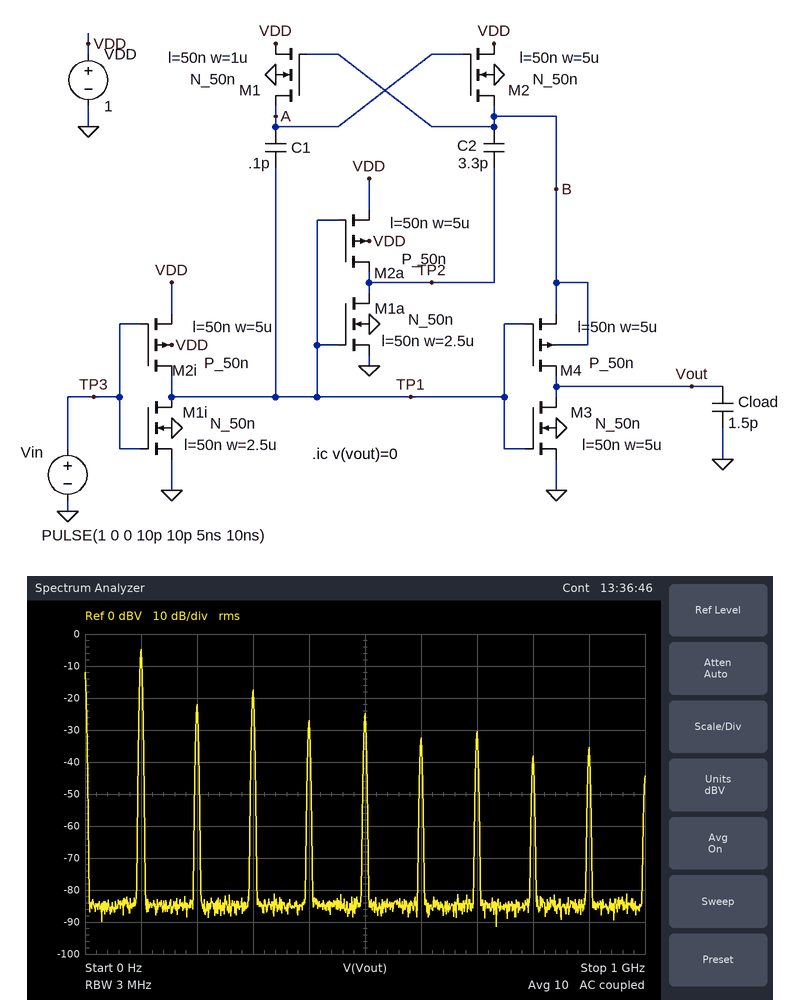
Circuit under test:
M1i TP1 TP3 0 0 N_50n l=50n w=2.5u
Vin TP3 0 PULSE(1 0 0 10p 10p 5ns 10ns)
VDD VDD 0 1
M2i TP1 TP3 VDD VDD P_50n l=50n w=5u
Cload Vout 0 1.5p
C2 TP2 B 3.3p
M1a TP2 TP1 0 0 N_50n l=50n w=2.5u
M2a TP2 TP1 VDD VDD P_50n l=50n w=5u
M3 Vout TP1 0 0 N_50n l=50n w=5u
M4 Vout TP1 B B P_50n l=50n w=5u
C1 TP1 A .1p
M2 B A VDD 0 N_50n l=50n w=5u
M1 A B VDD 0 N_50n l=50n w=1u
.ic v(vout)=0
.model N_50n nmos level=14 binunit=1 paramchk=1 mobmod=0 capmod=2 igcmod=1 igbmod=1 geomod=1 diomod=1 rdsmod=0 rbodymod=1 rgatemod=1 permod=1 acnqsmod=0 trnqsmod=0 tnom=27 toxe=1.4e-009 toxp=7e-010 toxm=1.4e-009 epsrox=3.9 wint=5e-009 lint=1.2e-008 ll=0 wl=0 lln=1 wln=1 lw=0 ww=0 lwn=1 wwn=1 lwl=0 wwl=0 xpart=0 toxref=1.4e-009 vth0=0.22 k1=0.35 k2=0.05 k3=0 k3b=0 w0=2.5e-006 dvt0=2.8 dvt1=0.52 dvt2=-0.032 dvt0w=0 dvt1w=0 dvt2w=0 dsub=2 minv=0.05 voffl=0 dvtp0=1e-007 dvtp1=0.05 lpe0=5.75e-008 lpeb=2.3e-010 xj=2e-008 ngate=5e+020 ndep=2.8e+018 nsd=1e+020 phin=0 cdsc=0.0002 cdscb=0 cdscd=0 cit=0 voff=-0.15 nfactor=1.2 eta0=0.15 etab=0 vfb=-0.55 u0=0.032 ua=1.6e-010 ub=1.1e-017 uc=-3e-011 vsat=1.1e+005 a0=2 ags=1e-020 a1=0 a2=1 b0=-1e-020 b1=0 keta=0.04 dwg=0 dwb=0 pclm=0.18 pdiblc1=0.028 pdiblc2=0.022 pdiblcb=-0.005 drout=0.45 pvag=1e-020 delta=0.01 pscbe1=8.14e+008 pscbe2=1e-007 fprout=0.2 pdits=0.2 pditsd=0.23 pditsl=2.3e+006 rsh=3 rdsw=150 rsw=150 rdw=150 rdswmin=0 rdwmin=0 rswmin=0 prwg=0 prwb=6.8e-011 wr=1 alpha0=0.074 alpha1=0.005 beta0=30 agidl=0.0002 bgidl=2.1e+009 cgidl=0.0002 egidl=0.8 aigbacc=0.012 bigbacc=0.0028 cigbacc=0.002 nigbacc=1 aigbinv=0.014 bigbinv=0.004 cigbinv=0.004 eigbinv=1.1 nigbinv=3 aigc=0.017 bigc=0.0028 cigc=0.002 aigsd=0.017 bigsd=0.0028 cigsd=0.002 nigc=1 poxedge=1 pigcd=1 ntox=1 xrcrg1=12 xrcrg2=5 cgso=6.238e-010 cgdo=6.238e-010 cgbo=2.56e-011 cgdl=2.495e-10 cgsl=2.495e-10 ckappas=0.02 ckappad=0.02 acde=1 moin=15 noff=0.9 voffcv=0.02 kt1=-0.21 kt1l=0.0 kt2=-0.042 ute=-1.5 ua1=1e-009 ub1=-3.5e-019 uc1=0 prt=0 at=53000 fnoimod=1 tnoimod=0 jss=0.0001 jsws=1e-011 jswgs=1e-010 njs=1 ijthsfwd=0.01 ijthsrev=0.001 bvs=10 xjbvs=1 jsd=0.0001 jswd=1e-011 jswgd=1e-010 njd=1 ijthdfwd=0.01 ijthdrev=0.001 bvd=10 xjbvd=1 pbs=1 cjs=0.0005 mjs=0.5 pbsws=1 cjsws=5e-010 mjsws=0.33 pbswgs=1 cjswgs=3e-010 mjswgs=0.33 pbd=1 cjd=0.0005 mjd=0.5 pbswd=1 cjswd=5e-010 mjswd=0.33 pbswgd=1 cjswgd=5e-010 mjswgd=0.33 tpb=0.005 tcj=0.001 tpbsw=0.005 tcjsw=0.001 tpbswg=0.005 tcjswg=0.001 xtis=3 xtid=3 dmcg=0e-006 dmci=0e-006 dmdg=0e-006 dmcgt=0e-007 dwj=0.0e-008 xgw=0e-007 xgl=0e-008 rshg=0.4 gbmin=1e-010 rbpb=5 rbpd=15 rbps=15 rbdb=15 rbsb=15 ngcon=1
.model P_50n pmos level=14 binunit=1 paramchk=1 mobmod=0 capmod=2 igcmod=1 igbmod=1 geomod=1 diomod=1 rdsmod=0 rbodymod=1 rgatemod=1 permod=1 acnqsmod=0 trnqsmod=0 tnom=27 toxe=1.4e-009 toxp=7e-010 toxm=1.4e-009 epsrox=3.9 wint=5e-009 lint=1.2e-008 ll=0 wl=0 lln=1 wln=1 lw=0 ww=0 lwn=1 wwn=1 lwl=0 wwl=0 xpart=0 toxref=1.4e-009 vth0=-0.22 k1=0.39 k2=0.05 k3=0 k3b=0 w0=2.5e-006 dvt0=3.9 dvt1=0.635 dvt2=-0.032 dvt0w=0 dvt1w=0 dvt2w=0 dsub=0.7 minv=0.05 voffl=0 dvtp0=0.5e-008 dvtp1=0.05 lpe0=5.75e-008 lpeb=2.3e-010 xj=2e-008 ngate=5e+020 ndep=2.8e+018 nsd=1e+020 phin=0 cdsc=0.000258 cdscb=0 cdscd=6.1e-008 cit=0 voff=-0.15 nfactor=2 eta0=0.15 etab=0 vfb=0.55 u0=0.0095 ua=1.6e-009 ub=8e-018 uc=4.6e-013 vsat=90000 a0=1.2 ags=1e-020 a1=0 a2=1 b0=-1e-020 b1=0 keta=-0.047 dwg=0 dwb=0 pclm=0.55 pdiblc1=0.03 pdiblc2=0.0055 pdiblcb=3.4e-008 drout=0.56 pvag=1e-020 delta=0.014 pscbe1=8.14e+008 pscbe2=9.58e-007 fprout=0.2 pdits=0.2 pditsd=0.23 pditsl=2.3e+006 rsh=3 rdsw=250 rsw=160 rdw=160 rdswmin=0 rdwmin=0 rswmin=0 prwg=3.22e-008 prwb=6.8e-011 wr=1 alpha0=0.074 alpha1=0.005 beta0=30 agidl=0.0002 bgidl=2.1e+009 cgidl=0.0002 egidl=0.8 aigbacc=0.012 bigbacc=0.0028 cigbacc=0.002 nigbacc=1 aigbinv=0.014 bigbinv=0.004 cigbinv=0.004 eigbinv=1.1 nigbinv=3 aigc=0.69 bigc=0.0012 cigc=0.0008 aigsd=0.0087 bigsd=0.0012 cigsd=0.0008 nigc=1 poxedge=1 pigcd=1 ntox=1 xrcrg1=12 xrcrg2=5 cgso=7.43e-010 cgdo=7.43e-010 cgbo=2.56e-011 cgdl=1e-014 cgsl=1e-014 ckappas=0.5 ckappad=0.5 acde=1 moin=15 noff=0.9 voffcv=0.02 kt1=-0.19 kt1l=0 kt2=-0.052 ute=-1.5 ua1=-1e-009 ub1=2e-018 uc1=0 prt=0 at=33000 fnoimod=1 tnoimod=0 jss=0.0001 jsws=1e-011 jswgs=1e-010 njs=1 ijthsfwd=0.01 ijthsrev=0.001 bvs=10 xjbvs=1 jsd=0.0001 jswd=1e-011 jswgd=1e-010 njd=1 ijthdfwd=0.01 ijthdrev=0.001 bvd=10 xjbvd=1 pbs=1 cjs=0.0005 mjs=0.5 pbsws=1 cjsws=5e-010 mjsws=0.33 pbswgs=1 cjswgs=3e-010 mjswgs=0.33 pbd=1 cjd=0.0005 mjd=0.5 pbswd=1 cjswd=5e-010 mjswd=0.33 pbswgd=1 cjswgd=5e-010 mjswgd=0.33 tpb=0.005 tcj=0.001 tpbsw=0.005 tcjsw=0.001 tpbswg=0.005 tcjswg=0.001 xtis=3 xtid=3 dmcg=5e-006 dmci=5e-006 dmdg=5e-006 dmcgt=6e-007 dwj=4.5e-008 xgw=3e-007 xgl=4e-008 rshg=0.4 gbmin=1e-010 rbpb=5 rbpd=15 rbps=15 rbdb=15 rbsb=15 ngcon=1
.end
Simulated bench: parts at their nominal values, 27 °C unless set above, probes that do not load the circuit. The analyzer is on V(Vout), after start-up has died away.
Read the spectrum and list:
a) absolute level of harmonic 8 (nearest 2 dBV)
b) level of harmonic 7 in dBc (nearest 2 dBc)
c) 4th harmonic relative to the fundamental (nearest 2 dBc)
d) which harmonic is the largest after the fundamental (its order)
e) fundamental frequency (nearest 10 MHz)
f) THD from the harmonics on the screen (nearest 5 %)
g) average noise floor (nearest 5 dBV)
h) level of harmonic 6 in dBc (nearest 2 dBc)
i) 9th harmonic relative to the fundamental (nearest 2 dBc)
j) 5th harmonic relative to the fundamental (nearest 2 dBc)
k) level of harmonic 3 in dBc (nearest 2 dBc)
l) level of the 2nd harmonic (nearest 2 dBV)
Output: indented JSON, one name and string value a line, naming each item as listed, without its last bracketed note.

{
  "absolute level of harmonic 8": "-38 dBV",
  "level of harmonic 7 in dBc": "-26 dBc",
  "4th harmonic relative to the fundamental": "-22 dBc",
  "which harmonic is the largest after the fundamental": "3",
  "fundamental frequency": "100 MHz",
  "THD from the harmonics on the screen": "30 %",
  "average noise floor": "-85 dBV",
  "level of harmonic 6 in dBc": "-28 dBc",
  "9th harmonic relative to the fundamental": "-30 dBc",
  "5th harmonic relative to the fundamental": "-20 dBc",
  "level of harmonic 3 in dBc": "-12 dBc",
  "level of the 2nd harmonic": "-22 dBV"
}
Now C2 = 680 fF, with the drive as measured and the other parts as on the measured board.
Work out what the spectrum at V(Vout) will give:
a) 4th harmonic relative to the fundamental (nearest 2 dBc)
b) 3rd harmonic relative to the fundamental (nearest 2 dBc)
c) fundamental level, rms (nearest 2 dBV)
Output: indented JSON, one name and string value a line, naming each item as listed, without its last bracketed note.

{
  "4th harmonic relative to the fundamental": "-26 dBc",
  "3rd harmonic relative to the fundamental": "-10 dBc",
  "fundamental level, rms": "-12 dBV"
}
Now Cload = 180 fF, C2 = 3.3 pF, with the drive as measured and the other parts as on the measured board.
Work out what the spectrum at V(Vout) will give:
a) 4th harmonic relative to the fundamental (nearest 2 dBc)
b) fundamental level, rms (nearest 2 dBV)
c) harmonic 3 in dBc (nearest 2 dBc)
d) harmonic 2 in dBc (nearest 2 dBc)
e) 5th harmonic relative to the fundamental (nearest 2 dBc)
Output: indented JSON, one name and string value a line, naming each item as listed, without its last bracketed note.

{
  "4th harmonic relative to the fundamental": "-30 dBc",
  "fundamental level, rms": "-2 dBV",
  "harmonic 3 in dBc": "-10 dBc",
  "harmonic 2 in dBc": "-30 dBc",
  "5th harmonic relative to the fundamental": "-14 dBc"
}
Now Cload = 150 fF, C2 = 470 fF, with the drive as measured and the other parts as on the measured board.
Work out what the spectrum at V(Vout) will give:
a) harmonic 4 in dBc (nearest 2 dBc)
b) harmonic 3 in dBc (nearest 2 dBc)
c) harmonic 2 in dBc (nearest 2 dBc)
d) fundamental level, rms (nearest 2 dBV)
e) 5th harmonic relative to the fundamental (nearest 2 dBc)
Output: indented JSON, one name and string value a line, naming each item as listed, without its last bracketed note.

{
  "harmonic 4 in dBc": "-32 dBc",
  "harmonic 3 in dBc": "-10 dBc",
  "harmonic 2 in dBc": "-32 dBc",
  "fundamental level, rms": "-4 dBV",
  "5th harmonic relative to the fundamental": "-14 dBc"
}
